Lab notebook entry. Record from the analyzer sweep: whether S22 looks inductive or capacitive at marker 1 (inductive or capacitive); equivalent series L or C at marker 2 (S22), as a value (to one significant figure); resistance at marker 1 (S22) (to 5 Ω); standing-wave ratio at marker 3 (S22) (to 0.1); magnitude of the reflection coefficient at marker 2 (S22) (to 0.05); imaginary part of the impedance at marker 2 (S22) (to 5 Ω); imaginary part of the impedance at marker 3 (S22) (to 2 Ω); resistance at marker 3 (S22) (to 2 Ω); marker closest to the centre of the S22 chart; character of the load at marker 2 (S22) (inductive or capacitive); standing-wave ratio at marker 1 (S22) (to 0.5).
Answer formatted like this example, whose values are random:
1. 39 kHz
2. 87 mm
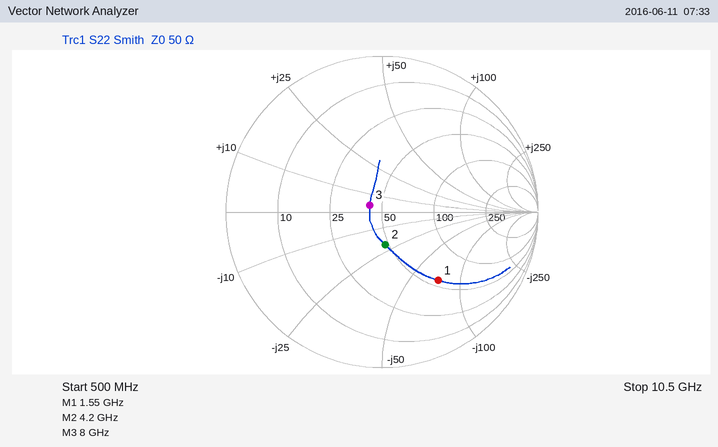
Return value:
1. capacitive
2. 2 pF
3. 55 Ω
4. 1.2
5. 0.20
6. -20 Ω
7. +4 Ω
8. 42 Ω
9. marker 3
10. capacitive
11. 3.5
